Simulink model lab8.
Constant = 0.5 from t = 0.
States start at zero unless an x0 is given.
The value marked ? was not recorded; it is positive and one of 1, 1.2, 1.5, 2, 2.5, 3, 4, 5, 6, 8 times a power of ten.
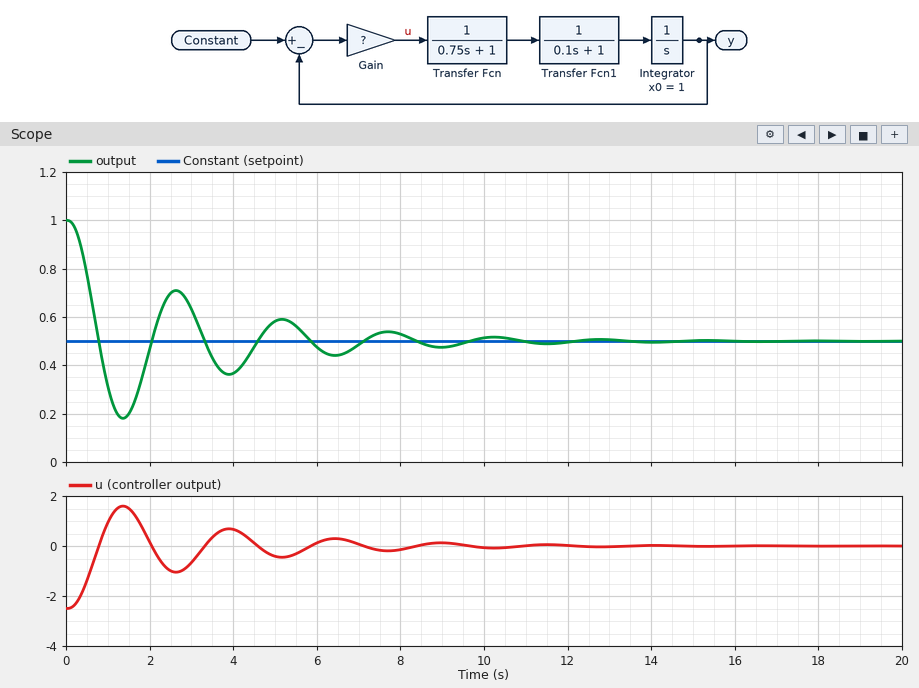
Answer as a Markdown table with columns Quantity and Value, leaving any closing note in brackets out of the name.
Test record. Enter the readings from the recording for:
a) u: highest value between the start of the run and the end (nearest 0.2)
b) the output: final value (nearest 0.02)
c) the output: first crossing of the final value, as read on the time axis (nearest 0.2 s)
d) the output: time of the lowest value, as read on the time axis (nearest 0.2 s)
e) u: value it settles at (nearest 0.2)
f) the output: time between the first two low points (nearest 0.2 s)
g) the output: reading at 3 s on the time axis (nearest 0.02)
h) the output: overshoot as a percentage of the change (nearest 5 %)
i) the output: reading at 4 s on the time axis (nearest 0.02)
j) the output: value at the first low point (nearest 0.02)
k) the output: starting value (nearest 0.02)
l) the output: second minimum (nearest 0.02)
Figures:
| Quantity | Value |
|---|---|
| u: highest value between the start of the run and the end | 1.6 |
| the output: final value | 0.50 |
| the output: first crossing of the final value, as read on the time axis | 0.8 s |
| the output: time of the lowest value, as read on the time axis | 1.4 s |
| u: value it settles at | 0.0 |
| the output: time between the first two low points | 2.6 s |
| the output: reading at 3 s on the time axis | 0.64 |
| the output: overshoot as a percentage of the change | 65 % |
| the output: reading at 4 s on the time axis | 0.36 |
| the output: value at the first low point | 0.18 |
| the output: starting value | 1.00 |
| the output: second minimum | 0.36 |
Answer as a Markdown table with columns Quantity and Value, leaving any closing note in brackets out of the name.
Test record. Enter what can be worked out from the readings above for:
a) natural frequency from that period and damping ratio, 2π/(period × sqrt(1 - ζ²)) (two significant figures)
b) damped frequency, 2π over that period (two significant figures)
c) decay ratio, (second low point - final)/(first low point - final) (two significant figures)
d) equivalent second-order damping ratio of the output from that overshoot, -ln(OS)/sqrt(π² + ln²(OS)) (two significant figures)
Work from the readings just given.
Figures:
| Quantity | Value |
|---|---|
| natural frequency from that period and damping ratio, 2π/(period × sqrt(1 - ζ²)) | 2.4 rad/s |
| damped frequency, 2π over that period | 2.4 rad/s |
| decay ratio, (second low point - final)/(first low point - final) | 0.44 |
| equivalent second-order damping ratio of the output from that overshoot, -ln(OS)/sqrt(π² + ln²(OS)) | 0.14 |
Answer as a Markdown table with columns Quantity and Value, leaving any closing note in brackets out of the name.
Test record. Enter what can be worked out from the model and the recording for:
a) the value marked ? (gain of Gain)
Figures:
| Quantity | Value |
|---|---|
| the value marked ? | 5 |
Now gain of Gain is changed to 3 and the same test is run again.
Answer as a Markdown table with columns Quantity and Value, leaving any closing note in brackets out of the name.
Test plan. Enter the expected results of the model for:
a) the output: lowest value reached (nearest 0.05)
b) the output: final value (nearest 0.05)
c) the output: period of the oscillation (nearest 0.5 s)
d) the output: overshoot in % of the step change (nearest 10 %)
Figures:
| Quantity | Value |
|---|---|
| the output: lowest value reached | 0.25 |
| the output: final value | 0.50 |
| the output: period of the oscillation | 3.5 s |
| the output: overshoot in % of the step change | 50 % |
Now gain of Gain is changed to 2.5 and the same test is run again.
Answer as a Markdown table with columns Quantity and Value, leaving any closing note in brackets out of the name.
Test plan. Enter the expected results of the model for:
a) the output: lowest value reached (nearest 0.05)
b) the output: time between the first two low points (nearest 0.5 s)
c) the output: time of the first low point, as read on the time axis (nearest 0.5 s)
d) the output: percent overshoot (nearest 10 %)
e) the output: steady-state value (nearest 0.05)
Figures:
| Quantity | Value |
|---|---|
| the output: lowest value reached | 0.30 |
| the output: time between the first two low points | 3.5 s |
| the output: time of the first low point, as read on the time axis | 2.0 s |
| the output: percent overshoot | 40 % |
| the output: steady-state value | 0.50 |
